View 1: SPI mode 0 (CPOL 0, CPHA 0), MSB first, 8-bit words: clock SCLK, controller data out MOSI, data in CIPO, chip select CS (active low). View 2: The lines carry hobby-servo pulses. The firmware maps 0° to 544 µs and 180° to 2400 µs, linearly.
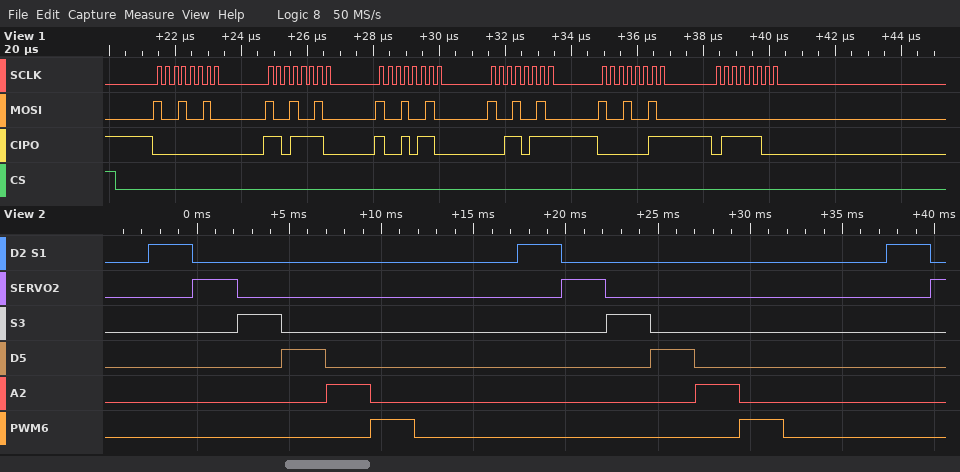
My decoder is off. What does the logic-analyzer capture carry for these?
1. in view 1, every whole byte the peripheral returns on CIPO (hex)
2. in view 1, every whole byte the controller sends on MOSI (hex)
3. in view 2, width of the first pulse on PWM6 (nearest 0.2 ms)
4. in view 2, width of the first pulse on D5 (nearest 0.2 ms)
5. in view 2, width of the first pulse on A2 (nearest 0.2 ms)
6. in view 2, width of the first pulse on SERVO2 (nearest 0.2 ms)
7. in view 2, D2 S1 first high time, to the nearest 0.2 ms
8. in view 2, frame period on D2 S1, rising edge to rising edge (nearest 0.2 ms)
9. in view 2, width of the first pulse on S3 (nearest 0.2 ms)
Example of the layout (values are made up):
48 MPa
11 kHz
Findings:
00 DE 96 37 03 7C
92 92 92 92 92 00
2.4 ms
2.4 ms
2.4 ms
2.4 ms
2.4 ms
20.0 ms
2.4 ms
